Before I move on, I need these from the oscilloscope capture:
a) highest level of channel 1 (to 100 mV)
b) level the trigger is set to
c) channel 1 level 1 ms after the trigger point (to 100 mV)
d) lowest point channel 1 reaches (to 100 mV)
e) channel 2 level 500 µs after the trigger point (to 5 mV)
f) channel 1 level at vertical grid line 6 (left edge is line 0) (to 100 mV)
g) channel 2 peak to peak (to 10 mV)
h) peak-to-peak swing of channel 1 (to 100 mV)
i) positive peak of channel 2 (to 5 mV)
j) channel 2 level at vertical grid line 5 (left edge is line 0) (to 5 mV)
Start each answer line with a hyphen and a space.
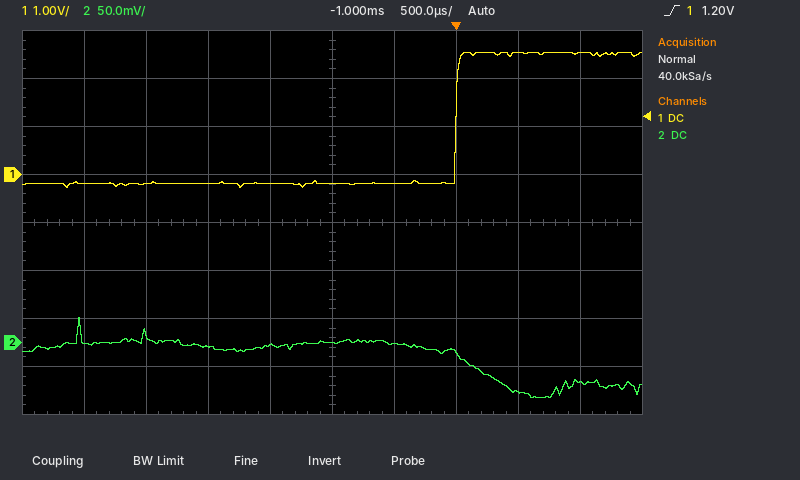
- 2.5 V
- 1.20 V
- 2.5 V
- -300 mV
- -50 mV
- -200 mV
- 80 mV
- 2.8 V
- 25 mV
- 0 mV
